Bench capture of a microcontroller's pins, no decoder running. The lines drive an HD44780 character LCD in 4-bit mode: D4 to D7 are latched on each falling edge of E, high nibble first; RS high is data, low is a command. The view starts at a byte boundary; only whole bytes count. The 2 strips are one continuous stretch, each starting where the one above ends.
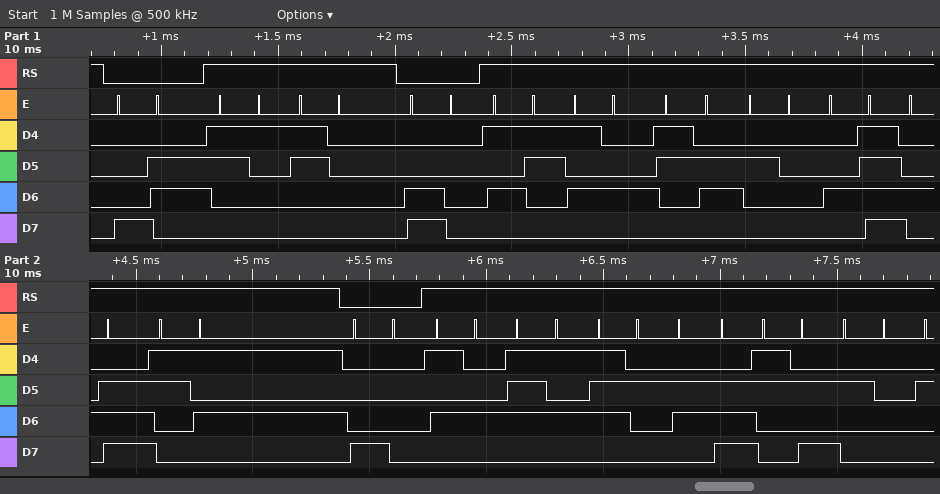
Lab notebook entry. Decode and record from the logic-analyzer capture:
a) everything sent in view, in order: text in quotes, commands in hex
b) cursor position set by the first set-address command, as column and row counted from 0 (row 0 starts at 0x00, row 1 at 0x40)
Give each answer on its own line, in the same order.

0x86 "10" 0xC0 "ST6 ON5" 0x80 "Turn: "
column 6, row 0
